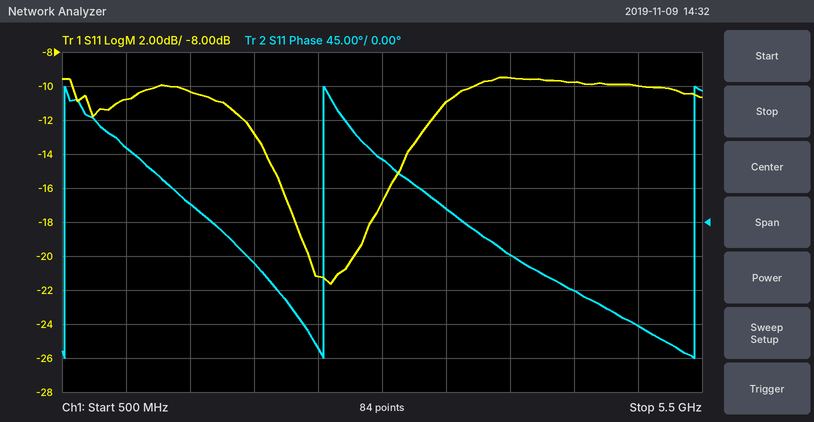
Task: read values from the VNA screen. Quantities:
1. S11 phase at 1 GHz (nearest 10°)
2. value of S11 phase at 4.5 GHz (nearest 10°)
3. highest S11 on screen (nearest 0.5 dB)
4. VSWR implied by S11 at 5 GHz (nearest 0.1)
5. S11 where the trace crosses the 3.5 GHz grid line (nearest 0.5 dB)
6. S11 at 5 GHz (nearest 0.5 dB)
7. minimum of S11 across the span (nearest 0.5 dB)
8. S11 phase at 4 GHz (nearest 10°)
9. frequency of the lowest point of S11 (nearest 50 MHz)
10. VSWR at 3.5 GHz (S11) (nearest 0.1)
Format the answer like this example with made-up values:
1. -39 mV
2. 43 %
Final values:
1. 100°
2. -90°
3. -9.5 dB
4. 1.9
5. -11.0 dB
6. -10.0 dB
7. -21.5 dB
8. -40°
9. 2.60 GHz
10. 1.8
